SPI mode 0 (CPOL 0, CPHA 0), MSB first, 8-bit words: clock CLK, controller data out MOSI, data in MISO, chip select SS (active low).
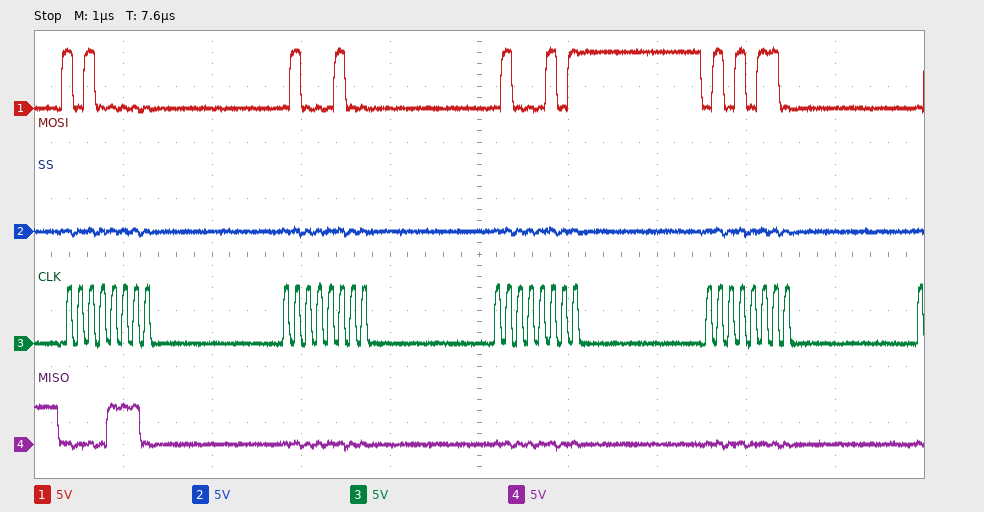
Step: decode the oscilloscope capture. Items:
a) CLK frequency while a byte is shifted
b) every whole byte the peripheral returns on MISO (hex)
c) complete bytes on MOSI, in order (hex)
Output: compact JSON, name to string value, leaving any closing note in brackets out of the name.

{"CLK frequency while a byte is shifted": "8 MHz", "every whole byte the peripheral returns on MISO": "0E 00 00 00", "complete bytes on MOSI, in order": "A0 44 45 56"}
